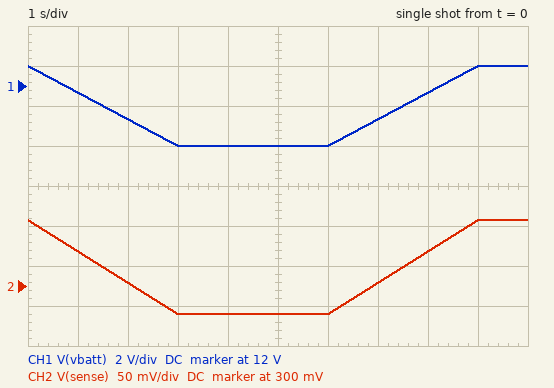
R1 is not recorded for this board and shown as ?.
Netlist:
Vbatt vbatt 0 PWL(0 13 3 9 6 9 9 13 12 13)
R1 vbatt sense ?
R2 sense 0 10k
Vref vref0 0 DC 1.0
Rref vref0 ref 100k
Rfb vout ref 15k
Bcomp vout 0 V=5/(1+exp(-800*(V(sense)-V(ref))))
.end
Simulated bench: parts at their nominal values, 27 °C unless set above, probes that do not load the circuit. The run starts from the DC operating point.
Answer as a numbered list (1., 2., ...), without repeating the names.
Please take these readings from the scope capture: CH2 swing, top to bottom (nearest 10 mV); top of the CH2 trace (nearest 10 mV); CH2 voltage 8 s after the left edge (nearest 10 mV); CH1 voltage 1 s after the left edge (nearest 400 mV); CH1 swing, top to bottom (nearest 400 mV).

1. 120 mV
2. 380 mV
3. 340 mV
4. 11.6 V
5. 4.0 V
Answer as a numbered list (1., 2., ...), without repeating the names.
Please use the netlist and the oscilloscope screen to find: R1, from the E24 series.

1. 330 kΩ
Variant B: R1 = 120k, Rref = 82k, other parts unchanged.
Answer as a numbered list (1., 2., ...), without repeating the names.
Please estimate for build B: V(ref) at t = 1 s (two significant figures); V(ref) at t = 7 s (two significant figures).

1. 900 mV
2. 800 mV
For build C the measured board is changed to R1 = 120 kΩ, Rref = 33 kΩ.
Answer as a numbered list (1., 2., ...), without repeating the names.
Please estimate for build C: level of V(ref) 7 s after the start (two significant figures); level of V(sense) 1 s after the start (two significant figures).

1. 800 mV
2. 900 mV
